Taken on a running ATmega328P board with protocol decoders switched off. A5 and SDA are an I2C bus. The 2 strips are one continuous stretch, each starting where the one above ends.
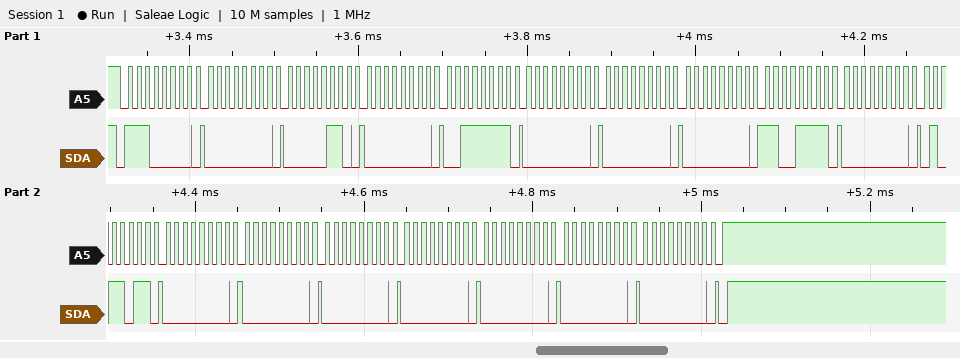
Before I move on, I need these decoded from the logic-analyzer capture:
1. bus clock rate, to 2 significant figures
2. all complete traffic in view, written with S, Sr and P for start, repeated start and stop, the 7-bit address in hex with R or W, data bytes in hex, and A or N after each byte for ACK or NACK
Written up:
100 kHz
S 70W A 00 A 06 A 00 A 3F A 00 A 00 A 00 A CF A 00 A 5B A 00 A 00 A 00 A 00 A 00 A 00 A 00 A P
